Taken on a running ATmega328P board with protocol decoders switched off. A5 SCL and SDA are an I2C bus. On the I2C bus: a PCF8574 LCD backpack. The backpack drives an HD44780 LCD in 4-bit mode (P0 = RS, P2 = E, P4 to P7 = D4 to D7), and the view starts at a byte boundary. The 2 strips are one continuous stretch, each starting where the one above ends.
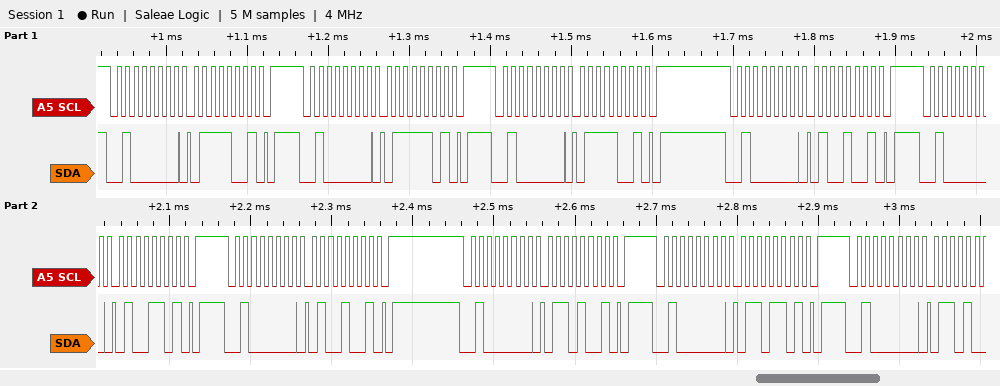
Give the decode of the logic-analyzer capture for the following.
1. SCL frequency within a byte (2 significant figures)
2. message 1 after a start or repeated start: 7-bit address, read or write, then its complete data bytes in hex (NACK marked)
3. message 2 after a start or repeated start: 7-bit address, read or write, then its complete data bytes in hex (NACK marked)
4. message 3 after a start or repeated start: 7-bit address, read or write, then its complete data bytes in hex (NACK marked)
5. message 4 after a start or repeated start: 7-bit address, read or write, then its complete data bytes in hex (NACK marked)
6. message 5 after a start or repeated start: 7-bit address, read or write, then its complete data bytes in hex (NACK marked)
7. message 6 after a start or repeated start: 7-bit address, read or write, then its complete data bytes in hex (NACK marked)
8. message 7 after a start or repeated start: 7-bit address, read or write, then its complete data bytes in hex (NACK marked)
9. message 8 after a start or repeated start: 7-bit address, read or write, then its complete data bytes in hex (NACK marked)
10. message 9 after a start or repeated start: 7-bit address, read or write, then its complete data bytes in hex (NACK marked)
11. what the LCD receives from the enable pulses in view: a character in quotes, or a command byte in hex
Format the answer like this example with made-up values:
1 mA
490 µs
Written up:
100 kHz
0x20 write: 79
0x20 write: 7D
0x20 write: 79
0x20 write: 49
0x20 write: 4D
0x20 write: 49
0x20 write: 69
0x20 write: 6D
0x20 write
't'
